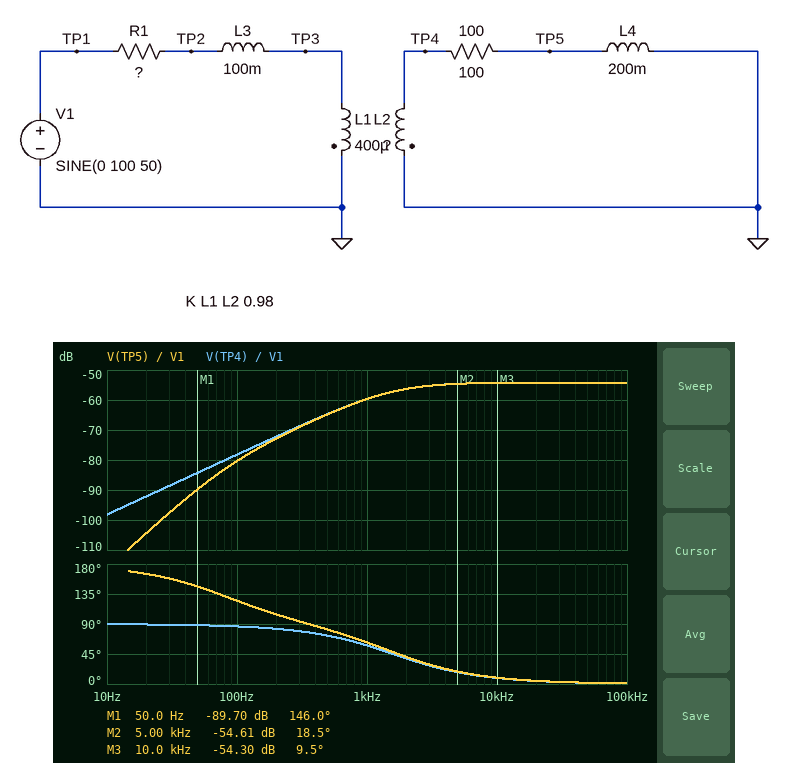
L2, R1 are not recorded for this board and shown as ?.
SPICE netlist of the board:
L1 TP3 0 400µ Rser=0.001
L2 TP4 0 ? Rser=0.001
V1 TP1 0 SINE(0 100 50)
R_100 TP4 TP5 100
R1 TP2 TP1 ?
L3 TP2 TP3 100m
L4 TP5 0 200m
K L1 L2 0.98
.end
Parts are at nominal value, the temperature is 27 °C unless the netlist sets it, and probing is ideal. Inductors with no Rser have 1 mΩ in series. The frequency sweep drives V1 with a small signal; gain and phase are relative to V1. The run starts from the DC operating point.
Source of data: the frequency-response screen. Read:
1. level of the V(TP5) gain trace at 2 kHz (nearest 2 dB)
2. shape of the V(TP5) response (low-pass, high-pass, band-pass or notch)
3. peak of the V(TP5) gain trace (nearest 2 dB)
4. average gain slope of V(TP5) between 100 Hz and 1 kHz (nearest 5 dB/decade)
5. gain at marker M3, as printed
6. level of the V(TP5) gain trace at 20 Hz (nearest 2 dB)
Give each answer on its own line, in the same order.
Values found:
-56 dB
high-pass
-54 dB
20 dB/decade
-54.30 dB
-104 dB
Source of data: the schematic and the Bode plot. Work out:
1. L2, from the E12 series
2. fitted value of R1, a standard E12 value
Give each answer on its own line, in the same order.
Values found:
100 µH
1 kΩ
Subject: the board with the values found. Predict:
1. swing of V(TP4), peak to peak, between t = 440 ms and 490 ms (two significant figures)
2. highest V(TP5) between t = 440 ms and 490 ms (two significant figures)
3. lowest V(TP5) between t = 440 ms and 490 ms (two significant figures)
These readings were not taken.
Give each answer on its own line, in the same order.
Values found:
12 mV
3.3 mV
-3.3 mV
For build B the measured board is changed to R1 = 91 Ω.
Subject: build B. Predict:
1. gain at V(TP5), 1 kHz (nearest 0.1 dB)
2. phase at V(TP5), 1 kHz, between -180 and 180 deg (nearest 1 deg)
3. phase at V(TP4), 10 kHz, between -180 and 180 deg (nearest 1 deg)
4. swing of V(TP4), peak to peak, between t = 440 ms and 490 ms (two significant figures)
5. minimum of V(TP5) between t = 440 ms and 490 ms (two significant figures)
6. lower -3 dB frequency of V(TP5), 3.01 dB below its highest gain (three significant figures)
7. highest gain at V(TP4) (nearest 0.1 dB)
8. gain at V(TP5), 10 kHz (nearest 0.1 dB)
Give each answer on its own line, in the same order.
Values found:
-54.3 dB
13 deg
1 deg
130 mV
-34 mV
177 Hz
-54.2 dB
-54.2 dB
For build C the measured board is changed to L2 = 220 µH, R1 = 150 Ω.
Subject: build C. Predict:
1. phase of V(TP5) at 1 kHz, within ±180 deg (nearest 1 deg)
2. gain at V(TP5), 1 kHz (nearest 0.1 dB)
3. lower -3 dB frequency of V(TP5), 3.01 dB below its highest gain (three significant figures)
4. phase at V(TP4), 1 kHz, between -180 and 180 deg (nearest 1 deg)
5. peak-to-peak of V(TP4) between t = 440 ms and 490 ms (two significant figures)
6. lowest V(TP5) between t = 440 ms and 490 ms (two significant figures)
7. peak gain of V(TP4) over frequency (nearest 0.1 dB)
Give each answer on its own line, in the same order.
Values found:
18 deg
-51.0 dB
261 Hz
13 deg
120 mV
-32 mV
-50.8 dB
